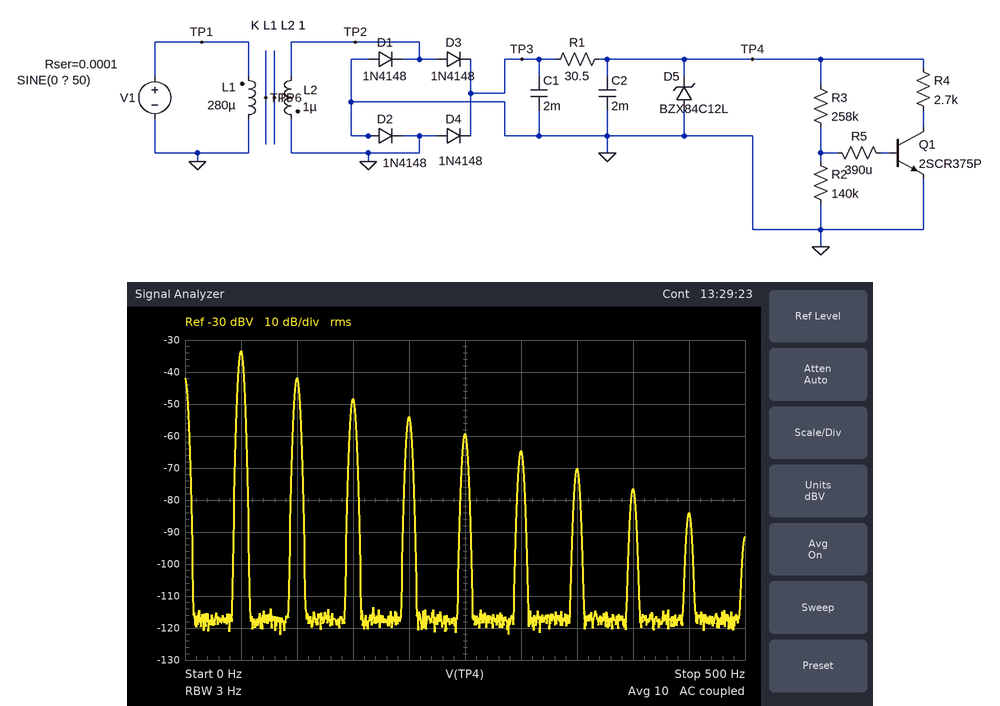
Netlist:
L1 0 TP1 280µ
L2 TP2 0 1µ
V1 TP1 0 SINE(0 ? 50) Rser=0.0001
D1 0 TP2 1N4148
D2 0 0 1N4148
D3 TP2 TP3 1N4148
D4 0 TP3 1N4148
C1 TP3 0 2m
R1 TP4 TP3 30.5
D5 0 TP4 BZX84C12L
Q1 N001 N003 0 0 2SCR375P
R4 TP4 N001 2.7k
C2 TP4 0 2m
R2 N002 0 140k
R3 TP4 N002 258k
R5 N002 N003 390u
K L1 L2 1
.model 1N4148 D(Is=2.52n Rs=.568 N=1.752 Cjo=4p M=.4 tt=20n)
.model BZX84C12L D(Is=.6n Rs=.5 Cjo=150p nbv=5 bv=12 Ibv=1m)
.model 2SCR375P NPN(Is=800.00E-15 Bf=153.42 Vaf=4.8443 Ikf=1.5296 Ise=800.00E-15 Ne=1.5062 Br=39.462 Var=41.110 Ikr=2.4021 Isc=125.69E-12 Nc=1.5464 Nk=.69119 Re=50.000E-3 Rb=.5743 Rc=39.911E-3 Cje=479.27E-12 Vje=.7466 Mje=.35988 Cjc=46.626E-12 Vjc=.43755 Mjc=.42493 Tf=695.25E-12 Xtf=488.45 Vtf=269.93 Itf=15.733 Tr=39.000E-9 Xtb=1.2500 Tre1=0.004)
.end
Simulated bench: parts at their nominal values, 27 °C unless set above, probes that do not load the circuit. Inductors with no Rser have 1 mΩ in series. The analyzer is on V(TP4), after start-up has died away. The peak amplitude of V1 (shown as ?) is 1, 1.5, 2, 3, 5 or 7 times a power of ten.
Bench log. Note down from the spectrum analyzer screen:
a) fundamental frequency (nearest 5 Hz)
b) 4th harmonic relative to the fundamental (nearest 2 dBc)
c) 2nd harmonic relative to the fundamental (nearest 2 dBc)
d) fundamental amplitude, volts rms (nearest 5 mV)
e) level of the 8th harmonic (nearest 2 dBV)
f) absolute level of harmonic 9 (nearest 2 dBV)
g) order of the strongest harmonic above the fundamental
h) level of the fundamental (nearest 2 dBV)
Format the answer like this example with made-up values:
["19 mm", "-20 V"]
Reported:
["50 Hz", "-20 dBc", "-8 dBc", "20 mV", "-76 dBV", "-84 dBV", "2", "-34 dBV"]
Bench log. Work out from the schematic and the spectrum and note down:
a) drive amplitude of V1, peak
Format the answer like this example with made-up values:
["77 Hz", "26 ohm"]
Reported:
["500 V"]
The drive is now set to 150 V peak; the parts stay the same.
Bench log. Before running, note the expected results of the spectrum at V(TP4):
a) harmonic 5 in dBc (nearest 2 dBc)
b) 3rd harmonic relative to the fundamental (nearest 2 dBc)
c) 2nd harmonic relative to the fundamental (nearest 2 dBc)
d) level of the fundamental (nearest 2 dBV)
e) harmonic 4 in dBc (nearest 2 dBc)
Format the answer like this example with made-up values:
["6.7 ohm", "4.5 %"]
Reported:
["-28 dBc", "-20 dBc", "-12 dBc", "-70 dBV", "-24 dBc"]
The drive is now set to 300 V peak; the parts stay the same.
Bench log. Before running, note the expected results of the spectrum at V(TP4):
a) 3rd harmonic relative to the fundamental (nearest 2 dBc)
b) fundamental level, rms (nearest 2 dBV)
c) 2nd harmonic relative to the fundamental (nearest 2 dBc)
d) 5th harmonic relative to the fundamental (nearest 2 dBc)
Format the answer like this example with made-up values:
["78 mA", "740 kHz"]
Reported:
["-18 dBc", "-40 dBV", "-10 dBc", "-28 dBc"]
